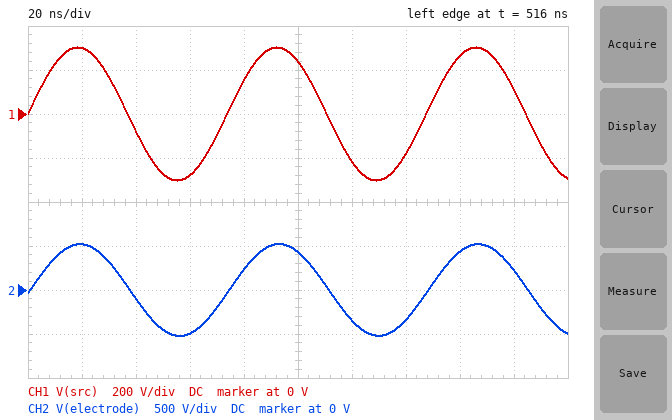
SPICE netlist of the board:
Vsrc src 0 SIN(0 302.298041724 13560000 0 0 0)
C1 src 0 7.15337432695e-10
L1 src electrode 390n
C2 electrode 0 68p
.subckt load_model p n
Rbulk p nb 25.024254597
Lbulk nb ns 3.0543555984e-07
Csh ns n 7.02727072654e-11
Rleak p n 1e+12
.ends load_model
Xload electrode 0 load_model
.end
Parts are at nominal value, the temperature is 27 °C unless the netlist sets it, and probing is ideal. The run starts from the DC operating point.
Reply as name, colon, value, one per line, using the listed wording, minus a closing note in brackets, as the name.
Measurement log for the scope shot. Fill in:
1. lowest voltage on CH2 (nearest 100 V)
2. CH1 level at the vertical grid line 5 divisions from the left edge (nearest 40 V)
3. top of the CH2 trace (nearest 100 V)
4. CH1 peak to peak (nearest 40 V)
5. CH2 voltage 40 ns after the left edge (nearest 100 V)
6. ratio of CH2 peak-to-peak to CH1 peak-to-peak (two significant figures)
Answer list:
lowest voltage on CH2: -500 V
CH1 level at the vertical grid line 5 divisions from the left edge: 240 V
top of the CH2 trace: 500 V
CH1 peak to peak: 600 V
CH2 voltage 40 ns after the left edge: -100 V
ratio of CH2 peak-to-peak to CH1 peak-to-peak: 1.7
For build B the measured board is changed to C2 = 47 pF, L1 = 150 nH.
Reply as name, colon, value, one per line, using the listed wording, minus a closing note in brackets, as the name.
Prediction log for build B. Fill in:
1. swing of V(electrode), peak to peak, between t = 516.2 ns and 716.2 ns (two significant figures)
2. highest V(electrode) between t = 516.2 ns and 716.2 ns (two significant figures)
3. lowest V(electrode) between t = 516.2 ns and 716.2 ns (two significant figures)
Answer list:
swing of V(electrode), peak to peak, between t = 516.2 ns and 716.2 ns: 700 V
highest V(electrode) between t = 516.2 ns and 716.2 ns: 350 V
lowest V(electrode) between t = 516.2 ns and 716.2 ns: -350 V
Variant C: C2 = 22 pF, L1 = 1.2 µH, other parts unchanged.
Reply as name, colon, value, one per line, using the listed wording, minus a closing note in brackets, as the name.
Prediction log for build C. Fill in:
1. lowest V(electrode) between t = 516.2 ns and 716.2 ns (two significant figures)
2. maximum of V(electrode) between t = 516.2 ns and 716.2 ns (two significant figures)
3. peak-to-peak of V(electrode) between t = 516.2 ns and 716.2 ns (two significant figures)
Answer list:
lowest V(electrode) between t = 516.2 ns and 716.2 ns: -1.9 kV
maximum of V(electrode) between t = 516.2 ns and 716.2 ns: 1.9 kV
peak-to-peak of V(electrode) between t = 516.2 ns and 716.2 ns: 3.7 kV
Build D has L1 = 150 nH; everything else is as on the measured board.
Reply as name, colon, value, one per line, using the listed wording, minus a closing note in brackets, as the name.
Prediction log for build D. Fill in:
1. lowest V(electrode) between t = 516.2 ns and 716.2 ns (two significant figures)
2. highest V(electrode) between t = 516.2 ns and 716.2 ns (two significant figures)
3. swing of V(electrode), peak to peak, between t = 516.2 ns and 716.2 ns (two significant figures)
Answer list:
lowest V(electrode) between t = 516.2 ns and 716.2 ns: -360 V
highest V(electrode) between t = 516.2 ns and 716.2 ns: 360 V
swing of V(electrode), peak to peak, between t = 516.2 ns and 716.2 ns: 720 V
